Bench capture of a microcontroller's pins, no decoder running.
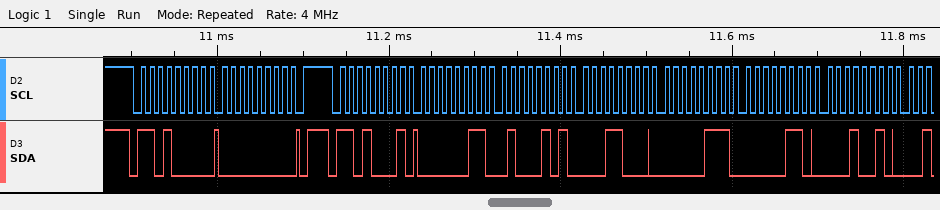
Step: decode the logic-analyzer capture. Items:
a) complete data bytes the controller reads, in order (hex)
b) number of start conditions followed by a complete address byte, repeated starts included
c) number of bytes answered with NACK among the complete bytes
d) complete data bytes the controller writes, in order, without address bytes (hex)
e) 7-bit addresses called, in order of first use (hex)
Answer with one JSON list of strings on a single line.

["03 45 18 07 06 12", "2", "0", "00", "0x68"]
